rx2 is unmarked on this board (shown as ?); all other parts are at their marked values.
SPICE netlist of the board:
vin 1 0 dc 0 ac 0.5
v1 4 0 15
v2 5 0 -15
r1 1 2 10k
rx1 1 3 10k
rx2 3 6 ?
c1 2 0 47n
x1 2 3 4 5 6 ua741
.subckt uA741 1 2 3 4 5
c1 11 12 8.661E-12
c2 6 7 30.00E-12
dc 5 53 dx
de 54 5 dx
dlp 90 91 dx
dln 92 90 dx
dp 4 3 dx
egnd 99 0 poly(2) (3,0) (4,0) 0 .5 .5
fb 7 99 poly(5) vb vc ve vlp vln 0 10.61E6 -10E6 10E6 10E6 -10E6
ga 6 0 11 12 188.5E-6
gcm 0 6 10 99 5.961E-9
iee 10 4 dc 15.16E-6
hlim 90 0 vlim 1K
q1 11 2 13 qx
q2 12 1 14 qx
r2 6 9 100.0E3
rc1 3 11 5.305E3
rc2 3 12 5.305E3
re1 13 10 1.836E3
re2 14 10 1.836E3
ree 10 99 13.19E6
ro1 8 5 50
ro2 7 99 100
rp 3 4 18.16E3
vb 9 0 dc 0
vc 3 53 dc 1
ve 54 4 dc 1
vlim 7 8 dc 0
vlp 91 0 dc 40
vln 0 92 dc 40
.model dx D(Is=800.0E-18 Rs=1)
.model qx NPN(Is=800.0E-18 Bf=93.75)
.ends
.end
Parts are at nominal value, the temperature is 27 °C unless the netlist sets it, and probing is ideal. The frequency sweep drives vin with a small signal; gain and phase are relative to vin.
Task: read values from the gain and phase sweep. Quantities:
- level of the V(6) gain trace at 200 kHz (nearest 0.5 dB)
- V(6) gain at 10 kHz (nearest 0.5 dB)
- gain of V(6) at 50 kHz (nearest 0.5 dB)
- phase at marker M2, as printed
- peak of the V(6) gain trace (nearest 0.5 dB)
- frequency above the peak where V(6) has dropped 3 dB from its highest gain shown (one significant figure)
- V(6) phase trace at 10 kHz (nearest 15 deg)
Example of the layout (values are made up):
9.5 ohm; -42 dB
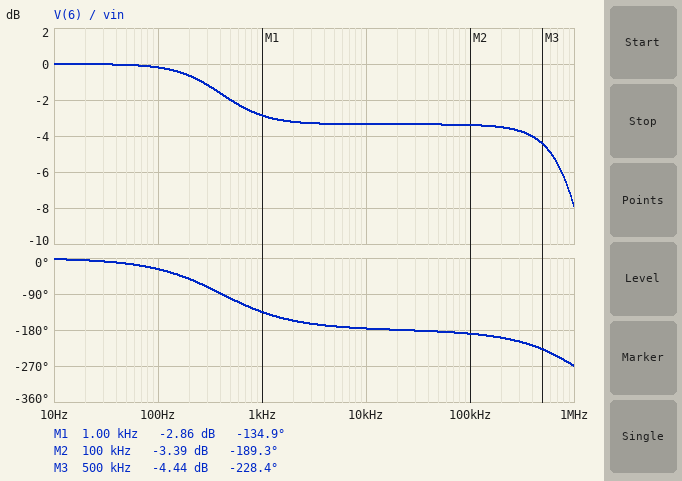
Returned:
-3.5 dB; -3.5 dB; -3.5 dB; -189.3 deg; 0 dB; 1 kHz; -180 deg
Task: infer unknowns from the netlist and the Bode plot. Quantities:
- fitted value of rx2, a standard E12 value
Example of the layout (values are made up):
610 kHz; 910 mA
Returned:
6.8 kΩ
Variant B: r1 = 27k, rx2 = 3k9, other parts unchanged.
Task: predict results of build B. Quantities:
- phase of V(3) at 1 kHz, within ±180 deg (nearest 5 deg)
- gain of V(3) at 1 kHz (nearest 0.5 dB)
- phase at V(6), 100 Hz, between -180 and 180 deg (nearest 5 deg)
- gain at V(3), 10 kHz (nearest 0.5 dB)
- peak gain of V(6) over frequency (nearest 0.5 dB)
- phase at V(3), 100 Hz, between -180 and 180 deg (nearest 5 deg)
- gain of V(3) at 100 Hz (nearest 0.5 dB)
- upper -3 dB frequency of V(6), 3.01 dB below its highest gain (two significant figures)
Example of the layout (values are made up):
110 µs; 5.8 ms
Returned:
-85 deg; -18.0 dB; -55 deg; -41.5 dB; 0 dB; -40 deg; -2.0 dB; 150 Hz
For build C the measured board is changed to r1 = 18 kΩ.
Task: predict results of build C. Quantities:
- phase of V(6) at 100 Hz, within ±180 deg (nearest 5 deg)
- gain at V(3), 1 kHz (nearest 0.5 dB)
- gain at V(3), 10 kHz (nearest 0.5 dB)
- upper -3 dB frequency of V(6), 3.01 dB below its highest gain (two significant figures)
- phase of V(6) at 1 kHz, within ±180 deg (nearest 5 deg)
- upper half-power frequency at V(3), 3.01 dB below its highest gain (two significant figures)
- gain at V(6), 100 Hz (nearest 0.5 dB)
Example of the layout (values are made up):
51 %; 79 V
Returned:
-50 deg; -14.5 dB; -38.5 dB; 690 Hz; -155 deg; 190 Hz; -0.5 dB
